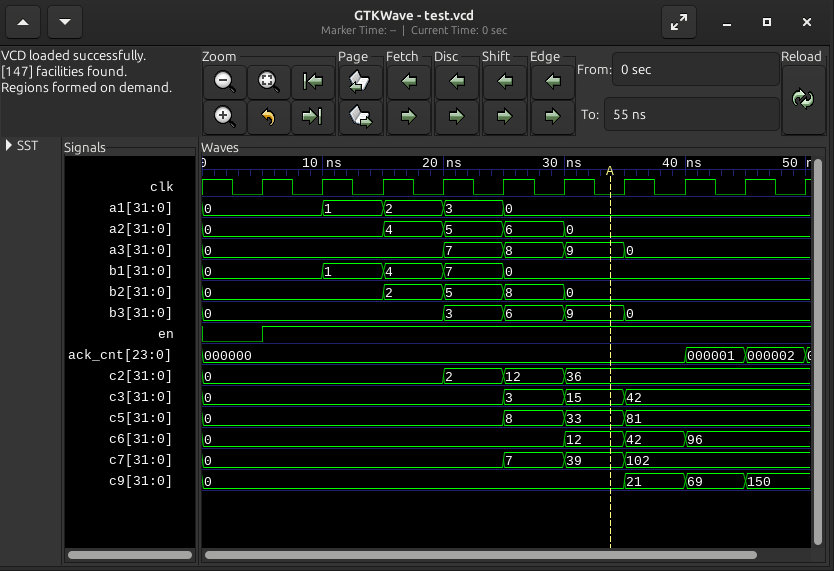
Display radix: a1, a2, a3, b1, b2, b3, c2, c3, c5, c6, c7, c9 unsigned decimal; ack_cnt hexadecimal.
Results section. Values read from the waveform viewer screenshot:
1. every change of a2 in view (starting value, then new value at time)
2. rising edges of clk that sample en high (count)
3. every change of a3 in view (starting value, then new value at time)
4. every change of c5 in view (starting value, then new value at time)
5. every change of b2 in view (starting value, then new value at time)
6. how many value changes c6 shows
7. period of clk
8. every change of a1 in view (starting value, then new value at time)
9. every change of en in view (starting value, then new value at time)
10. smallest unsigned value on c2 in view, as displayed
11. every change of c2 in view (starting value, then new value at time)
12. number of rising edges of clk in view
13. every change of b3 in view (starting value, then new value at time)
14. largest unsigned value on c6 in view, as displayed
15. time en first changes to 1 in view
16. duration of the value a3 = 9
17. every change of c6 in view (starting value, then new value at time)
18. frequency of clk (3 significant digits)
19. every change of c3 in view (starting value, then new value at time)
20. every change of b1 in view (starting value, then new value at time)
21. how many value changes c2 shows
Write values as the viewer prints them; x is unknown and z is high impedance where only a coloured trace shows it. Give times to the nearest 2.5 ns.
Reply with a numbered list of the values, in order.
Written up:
1. 0, 4 at 15 ns, 5 at 20 ns, 6 at 25 ns, 0 at 30 ns
2. 9
3. 0, 7 at 20 ns, 8 at 25 ns, 9 at 30 ns, 0 at 35 ns
4. 0, 8 at 25 ns, 33 at 30 ns, 81 at 35 ns
5. 0, 2 at 15 ns, 5 at 20 ns, 8 at 25 ns, 0 at 30 ns
6. 3
7. 5 ns
8. 0, 1 at 10 ns, 2 at 15 ns, 3 at 20 ns, 0 at 25 ns
9. 0, 1 at 5 ns
10. 0
11. 0, 2 at 20 ns, 12 at 25 ns, 36 at 30 ns
12. 10
13. 0, 3 at 20 ns, 6 at 25 ns, 9 at 30 ns, 0 at 35 ns
14. 96
15. 5 ns
16. 5 ns
17. 0, 12 at 30 ns, 42 at 35 ns, 96 at 40 ns
18. 200 MHz
19. 0, 3 at 25 ns, 15 at 30 ns, 42 at 35 ns
20. 0, 1 at 10 ns, 4 at 15 ns, 7 at 20 ns, 0 at 25 ns
21. 3
